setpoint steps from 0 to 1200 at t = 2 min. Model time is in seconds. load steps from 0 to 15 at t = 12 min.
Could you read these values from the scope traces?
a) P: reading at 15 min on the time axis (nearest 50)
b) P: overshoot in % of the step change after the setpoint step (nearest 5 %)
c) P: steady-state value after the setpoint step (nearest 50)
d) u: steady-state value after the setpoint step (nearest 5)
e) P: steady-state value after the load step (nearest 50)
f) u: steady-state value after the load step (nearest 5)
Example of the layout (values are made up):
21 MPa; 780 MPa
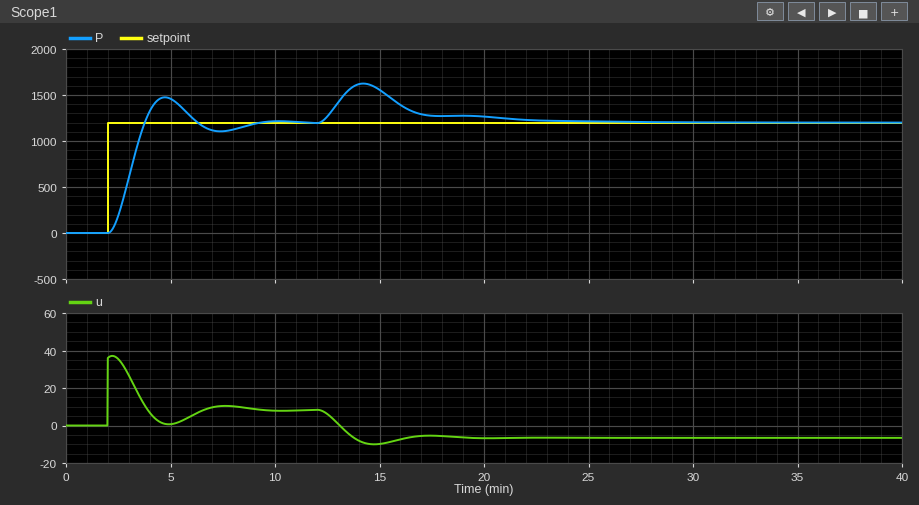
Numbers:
1550; 25 %; 1200; 10; 1200; -5
